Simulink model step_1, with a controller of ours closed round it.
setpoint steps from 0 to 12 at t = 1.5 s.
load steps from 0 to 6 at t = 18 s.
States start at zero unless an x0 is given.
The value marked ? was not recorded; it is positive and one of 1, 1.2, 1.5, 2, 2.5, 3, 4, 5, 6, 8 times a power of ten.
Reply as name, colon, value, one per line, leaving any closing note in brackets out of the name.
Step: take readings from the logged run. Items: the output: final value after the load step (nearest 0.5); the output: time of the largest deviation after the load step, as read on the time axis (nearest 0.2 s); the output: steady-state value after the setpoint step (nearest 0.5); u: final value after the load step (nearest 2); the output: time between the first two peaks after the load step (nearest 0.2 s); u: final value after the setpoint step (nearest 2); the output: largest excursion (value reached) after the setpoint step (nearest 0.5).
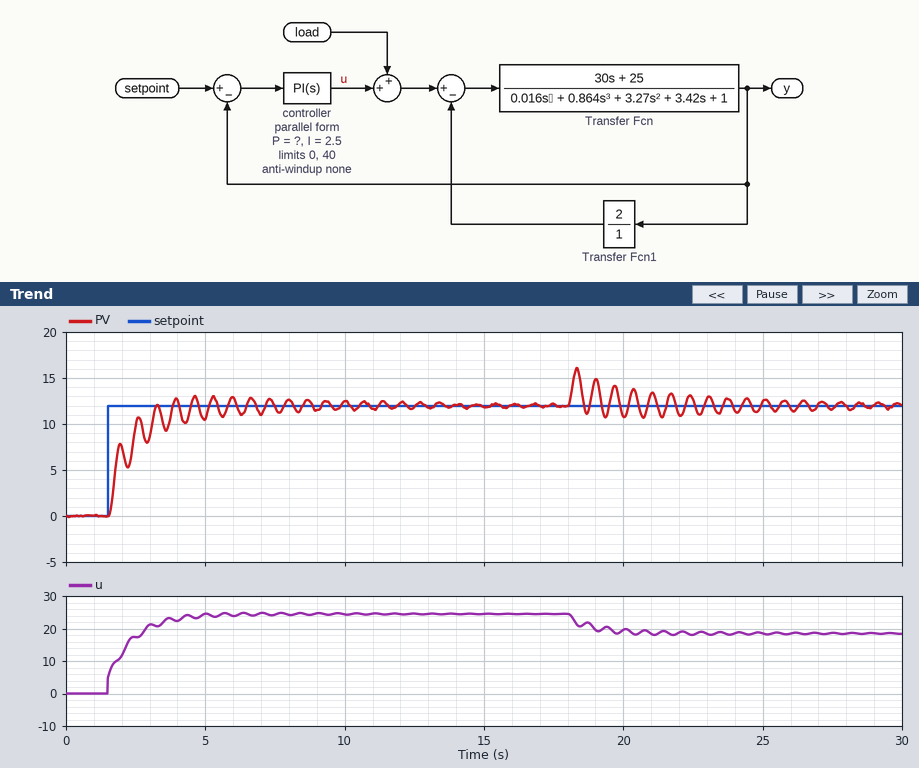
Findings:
the output: final value after the load step: 12.0
the output: time of the largest deviation after the load step, as read on the time axis: 18.4 s
the output: steady-state value after the setpoint step: 12.0
u: final value after the load step: 18
the output: time between the first two peaks after the load step: 0.6 s
u: final value after the setpoint step: 24
the output: largest excursion (value reached) after the setpoint step: 13.0
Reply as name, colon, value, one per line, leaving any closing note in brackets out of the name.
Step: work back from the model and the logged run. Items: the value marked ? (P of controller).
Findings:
the value marked ?: 0.4
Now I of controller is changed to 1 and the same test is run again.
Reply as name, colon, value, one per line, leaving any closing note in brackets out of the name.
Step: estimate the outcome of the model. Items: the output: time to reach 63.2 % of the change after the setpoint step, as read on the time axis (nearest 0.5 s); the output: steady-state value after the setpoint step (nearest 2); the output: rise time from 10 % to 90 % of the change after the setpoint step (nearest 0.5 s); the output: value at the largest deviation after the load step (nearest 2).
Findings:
the output: time to reach 63.2 % of the change after the setpoint step, as read on the time axis: 3.0 s
the output: steady-state value after the setpoint step: 12
the output: rise time from 10 % to 90 % of the change after the setpoint step: 5.0 s
the output: value at the largest deviation after the load step: 16
